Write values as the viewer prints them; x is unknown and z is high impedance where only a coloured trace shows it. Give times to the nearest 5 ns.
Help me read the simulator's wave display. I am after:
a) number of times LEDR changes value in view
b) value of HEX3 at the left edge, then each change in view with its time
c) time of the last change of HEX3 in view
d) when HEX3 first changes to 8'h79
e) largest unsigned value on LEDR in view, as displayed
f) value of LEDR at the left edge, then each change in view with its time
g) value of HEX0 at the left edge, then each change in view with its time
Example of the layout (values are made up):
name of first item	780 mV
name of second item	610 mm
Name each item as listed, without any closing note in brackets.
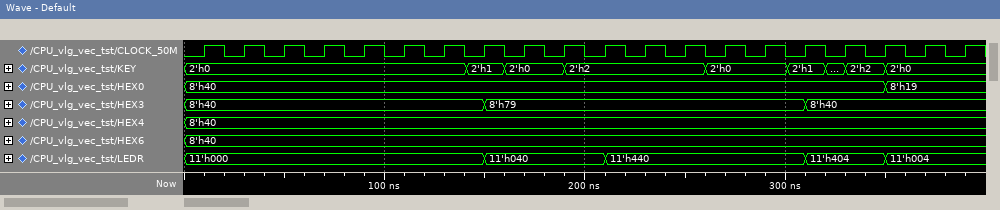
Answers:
number of times LEDR changes value in view	4
value of HEX3 at the left edge, then each change in view with its time	8'h40, 8'h79 at 150 ns, 8'h40 at 310 ns
time of the last change of HEX3 in view	310 ns
when HEX3 first changes to 8'h79	150 ns
largest unsigned value on LEDR in view, as displayed	11'h440
value of LEDR at the left edge, then each change in view with its time	11'h000, 11'h040 at 150 ns, 11'h440 at 210 ns, 11'h404 at 310 ns, 11'h004 at 350 ns
value of HEX0 at the left edge, then each change in view with its time	8'h40, 8'h19 at 350 ns
